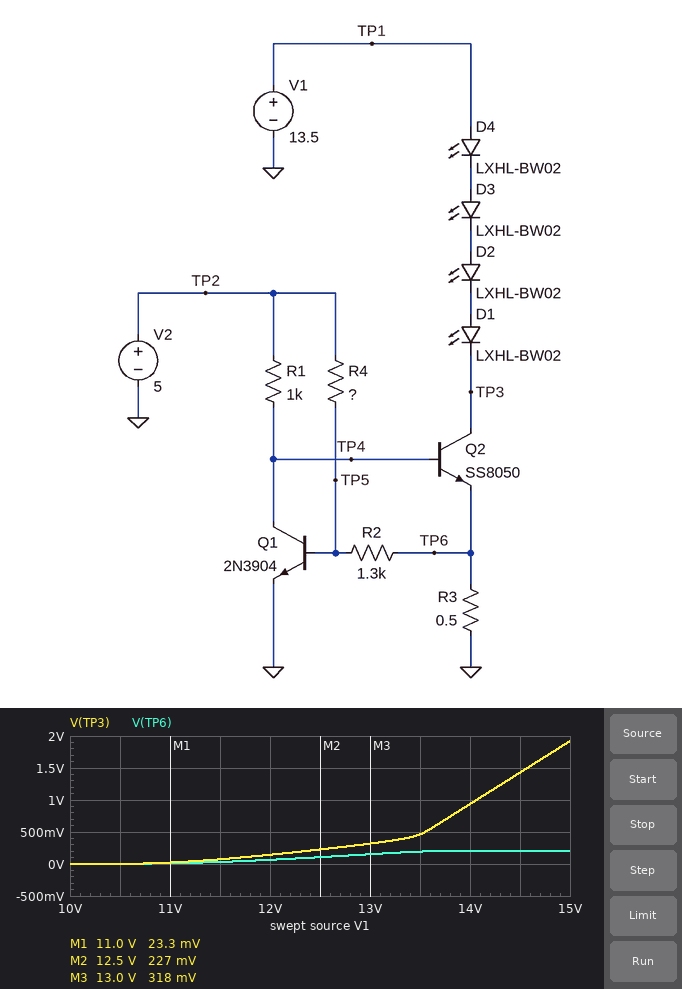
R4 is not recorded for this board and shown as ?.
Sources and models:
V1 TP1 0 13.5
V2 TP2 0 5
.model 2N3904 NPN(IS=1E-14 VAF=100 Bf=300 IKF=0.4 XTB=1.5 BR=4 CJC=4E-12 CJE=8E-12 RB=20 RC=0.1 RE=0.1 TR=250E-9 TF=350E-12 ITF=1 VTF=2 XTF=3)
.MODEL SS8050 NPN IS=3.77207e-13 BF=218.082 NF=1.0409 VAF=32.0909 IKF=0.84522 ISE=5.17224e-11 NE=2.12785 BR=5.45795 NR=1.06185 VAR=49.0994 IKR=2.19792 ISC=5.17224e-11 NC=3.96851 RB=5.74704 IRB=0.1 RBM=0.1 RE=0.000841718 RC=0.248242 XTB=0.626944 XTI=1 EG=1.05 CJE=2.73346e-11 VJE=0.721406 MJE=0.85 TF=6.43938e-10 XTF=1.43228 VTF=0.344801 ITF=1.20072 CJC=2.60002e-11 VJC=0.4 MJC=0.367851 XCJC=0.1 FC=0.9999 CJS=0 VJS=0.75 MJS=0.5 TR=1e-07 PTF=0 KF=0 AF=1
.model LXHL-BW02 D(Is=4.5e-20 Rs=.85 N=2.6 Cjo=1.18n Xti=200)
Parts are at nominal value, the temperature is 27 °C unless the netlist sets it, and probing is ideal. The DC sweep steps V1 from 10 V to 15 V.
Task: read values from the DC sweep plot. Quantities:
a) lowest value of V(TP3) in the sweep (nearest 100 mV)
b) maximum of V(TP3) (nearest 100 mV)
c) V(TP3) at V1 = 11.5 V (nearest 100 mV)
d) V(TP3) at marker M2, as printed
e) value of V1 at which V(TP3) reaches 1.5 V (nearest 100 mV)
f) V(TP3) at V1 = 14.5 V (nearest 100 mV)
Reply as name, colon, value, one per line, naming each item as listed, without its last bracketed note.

lowest value of V(TP3) in the sweep: 0 V
maximum of V(TP3): 1.9 V
V(TP3) at V1 = 11.5 V: 100 mV
V(TP3) at marker M2, as printed: 227 mV
value of V1 at which V(TP3) reaches 1.5 V: 14.6 V
V(TP3) at V1 = 14.5 V: 1.4 V
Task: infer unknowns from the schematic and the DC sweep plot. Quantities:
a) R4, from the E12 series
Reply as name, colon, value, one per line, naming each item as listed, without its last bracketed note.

R4, from the E12 series: 12 kΩ
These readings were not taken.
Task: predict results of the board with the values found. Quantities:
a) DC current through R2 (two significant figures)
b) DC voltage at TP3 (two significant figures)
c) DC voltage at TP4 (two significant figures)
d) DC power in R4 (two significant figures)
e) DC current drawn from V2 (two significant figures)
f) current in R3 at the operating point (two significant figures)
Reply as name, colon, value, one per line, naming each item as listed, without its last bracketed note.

DC current through R2: 360 µA
DC voltage at TP3: 460 mV
DC voltage at TP4: 970 mV
DC power in R4: 1.6 mW
DC current drawn from V2: 4.4 mA
current in R3 at the operating point: 390 mA
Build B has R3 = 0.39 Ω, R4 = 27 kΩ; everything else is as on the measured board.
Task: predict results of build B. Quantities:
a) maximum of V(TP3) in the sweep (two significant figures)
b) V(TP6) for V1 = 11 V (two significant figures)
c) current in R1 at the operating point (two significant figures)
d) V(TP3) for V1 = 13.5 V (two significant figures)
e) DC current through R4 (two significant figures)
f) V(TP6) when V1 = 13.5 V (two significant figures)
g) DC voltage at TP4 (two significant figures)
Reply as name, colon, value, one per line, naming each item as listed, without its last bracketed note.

maximum of V(TP3) in the sweep: 1.4 V
V(TP6) for V1 = 11 V: 9.1 mV
current in R1 at the operating point: 4.1 mA
V(TP3) for V1 = 13.5 V: 380 mV
DC current through R4: 170 µA
V(TP6) when V1 = 13.5 V: 160 mV
DC voltage at TP4: 940 mV
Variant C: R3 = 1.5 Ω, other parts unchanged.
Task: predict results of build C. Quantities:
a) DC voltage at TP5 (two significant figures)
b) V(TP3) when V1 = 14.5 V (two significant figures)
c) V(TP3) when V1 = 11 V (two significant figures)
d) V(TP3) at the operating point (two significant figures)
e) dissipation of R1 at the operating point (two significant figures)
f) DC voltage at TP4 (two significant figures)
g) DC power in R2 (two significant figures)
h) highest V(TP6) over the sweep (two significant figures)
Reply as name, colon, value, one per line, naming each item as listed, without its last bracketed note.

DC voltage at TP5: 690 mV
V(TP3) when V1 = 14.5 V: 2.5 V
V(TP3) when V1 = 11 V: 44 mV
V(TP3) at the operating point: 1.5 V
dissipation of R1 at the operating point: 16 mW
DC voltage at TP4: 960 mV
DC power in R2: 160 µW
highest V(TP6) over the sweep: 230 mV
